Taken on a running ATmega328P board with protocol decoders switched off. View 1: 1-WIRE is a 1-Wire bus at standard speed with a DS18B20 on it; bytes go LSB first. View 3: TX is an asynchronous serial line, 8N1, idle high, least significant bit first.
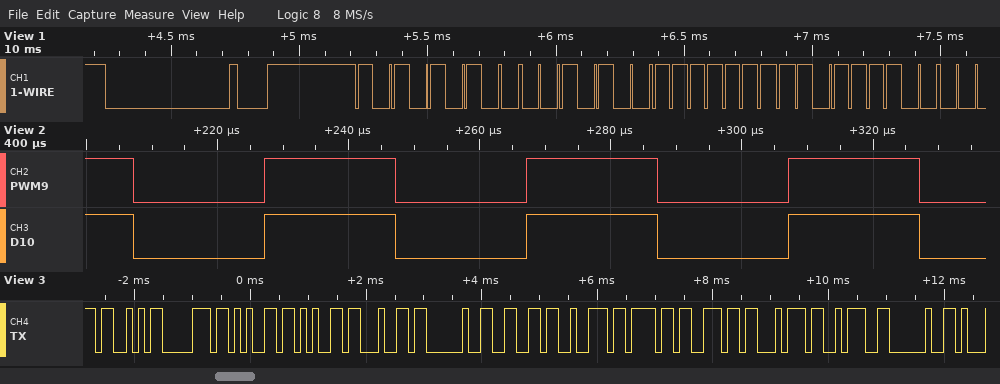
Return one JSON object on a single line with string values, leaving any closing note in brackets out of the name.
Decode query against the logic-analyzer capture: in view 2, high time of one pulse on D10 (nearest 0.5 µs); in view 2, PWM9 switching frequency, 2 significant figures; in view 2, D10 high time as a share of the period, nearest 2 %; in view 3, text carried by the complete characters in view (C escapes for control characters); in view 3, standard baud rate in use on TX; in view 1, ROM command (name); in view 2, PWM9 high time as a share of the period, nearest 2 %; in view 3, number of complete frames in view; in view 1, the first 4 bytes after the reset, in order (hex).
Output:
{"in view 2, high time of one pulse on D10": "20.0 µs", "in view 2, PWM9 switching frequency, 2 significant figures": "25 kHz", "in view 2, D10 high time as a share of the period, nearest 2 %": "50 %", "in view 3, text carried by the complete characters in view": "\"Speed front: \"", "in view 3, standard baud rate in use on TX": "9600 baud", "in view 1, ROM command": "Match ROM", "in view 2, PWM9 high time as a share of the period, nearest 2 %": "50 %", "in view 3, number of complete frames in view": "13", "in view 1, the first 4 bytes after the reset, in order": "55 28 FF 3D"}
